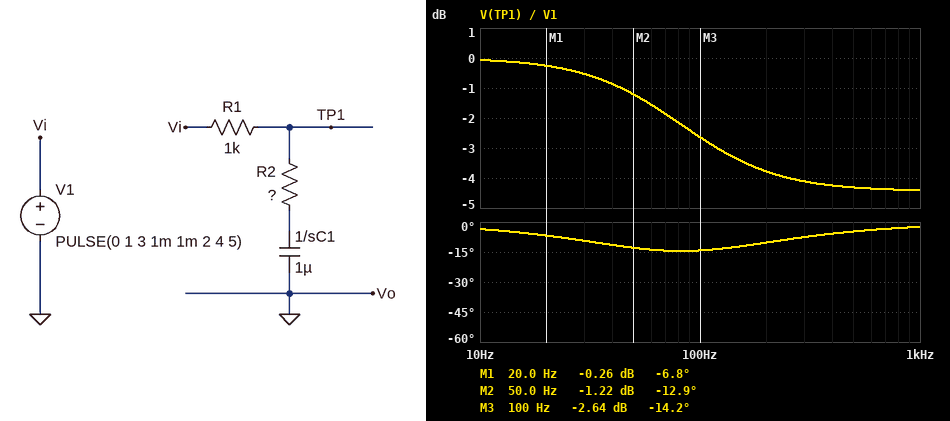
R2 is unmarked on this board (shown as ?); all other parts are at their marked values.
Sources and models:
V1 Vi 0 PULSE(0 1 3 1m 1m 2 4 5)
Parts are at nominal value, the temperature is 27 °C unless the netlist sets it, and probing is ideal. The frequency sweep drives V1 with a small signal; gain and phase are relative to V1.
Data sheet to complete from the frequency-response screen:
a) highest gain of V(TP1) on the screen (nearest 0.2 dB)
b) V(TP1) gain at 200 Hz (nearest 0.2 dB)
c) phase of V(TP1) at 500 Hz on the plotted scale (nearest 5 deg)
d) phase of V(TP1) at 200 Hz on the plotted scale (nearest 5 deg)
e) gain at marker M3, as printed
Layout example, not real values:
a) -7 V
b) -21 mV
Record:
a) 0 dB
b) -3.8 dB
c) -5 deg
d) -10 deg
e) -2.64 dB
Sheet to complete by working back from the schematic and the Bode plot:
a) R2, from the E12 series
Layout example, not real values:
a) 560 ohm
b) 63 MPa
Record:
a) 1.5 kΩ
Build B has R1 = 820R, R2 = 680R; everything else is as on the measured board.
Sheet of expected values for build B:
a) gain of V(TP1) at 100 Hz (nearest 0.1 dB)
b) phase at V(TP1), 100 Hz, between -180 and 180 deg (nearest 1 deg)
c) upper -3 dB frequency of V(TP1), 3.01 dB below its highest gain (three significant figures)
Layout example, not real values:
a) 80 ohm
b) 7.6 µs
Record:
a) -2.0 dB
b) -20 deg
c) 138 Hz
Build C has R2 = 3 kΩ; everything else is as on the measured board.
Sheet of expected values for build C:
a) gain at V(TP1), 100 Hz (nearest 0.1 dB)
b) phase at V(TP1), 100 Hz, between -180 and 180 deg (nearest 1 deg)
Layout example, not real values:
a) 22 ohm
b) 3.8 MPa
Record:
a) -2.1 dB
b) -6 deg
